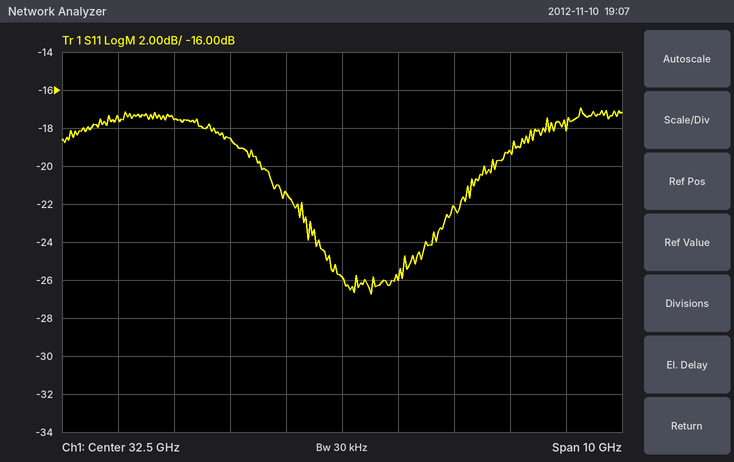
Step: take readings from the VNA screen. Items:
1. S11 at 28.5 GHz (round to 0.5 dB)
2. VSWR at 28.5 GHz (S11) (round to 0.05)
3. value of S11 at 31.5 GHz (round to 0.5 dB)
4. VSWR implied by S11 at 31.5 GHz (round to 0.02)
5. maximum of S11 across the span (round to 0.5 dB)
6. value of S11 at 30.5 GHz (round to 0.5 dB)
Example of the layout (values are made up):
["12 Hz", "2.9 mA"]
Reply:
["-17.5 dB", "1.30", "-21.5 dB", "1.18", "-17.0 dB", "-18.5 dB"]
